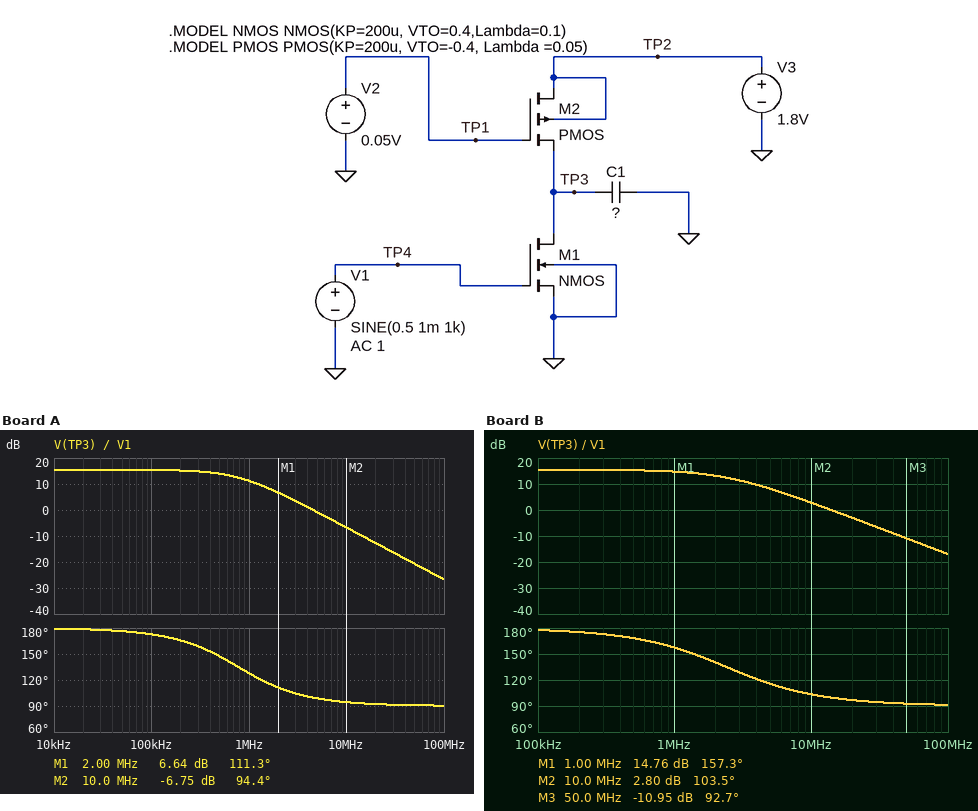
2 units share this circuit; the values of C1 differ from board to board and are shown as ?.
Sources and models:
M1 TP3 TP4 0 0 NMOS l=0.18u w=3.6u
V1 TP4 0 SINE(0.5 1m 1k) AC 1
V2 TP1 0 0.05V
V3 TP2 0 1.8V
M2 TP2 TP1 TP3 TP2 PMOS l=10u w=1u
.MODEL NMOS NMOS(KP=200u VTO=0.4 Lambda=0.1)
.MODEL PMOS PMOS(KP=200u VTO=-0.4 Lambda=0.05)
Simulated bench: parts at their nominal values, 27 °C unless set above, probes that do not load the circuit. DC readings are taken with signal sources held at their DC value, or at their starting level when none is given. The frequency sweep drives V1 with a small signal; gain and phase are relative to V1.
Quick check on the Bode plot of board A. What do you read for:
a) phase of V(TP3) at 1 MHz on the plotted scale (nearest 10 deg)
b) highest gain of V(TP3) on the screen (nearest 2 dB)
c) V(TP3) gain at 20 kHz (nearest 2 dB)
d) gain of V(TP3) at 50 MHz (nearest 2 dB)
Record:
130 deg
16 dB
16 dB
-20 dB
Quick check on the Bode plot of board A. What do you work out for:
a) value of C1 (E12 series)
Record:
12 pF
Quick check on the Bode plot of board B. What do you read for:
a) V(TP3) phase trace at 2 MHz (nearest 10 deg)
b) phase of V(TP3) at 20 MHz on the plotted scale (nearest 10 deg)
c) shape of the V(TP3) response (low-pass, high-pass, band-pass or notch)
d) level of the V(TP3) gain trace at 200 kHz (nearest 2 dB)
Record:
140 deg
100 deg
low-pass
16 dB
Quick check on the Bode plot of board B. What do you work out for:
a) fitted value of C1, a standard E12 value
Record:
3.9 pF
